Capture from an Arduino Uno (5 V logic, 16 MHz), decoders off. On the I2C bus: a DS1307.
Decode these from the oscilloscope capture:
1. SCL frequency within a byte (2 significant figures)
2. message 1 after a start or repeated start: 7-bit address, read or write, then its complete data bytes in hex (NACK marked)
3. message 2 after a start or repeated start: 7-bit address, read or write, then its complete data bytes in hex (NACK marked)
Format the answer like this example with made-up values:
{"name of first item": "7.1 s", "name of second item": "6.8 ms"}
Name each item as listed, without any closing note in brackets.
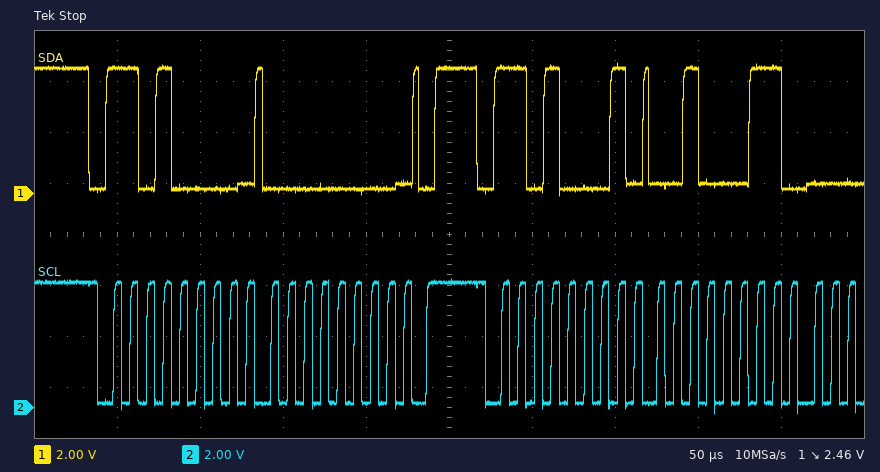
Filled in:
{"SCL frequency within a byte": "100 kHz", "message 1 after a start or repeated start: 7-bit address, read or write, then its complete data bytes in hex": "0x68 write: 00", "message 2 after a start or repeated start: 7-bit address, read or write, then its complete data bytes in hex": "0x68 read: 23"}
